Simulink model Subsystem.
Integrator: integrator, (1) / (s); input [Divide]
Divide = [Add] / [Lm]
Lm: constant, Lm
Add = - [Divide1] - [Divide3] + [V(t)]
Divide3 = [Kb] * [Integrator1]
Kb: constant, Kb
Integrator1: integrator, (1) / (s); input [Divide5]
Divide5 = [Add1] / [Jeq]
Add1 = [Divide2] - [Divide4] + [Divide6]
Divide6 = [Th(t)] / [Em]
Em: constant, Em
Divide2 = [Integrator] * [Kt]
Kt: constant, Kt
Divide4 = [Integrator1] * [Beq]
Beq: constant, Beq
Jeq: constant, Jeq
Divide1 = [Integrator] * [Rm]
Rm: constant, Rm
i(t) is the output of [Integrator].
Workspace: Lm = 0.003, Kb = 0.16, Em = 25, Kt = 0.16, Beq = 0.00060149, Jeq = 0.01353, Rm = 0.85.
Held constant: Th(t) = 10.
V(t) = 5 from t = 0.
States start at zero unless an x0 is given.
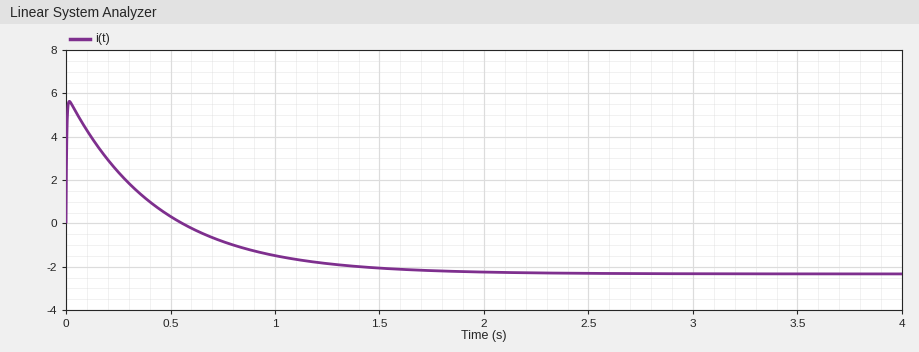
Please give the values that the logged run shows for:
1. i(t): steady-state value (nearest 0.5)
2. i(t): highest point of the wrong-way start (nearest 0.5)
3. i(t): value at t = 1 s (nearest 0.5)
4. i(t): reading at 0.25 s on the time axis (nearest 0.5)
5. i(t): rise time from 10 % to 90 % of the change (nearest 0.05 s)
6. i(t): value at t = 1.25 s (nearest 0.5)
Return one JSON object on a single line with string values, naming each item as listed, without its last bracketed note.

{"i(t): steady-state value": "-2.5", "i(t): highest point of the wrong-way start": "5.5", "i(t): value at t = 1 s": "-1.5", "i(t): reading at 0.25 s on the time axis": "2.5", "i(t): rise time from 10 % to 90 % of the change": "0.95 s", "i(t): value at t = 1.25 s": "-2.0"}
